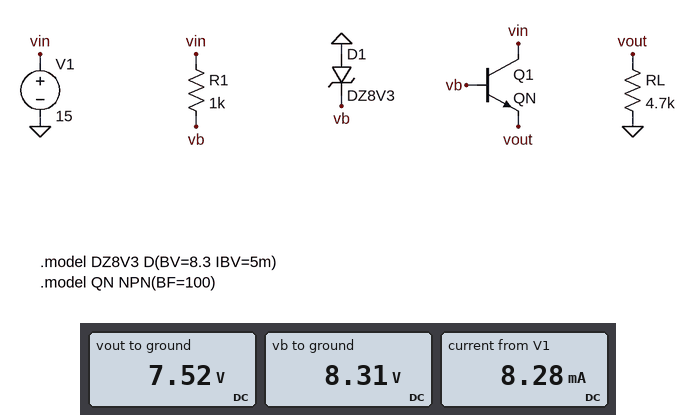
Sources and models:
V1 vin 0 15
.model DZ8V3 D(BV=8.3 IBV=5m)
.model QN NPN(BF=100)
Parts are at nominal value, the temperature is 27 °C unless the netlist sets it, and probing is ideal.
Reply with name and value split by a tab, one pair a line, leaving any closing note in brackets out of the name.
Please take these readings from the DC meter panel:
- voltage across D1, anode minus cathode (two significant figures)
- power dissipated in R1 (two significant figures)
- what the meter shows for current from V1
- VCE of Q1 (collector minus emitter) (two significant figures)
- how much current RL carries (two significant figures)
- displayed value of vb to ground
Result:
voltage across D1, anode minus cathode	-8.3 V
power dissipated in R1	45 mW
what the meter shows for current from V1	8.28 mA
VCE of Q1 (collector minus emitter)	7.5 V
how much current RL carries	1.6 mA
displayed value of vb to ground	8.31 V
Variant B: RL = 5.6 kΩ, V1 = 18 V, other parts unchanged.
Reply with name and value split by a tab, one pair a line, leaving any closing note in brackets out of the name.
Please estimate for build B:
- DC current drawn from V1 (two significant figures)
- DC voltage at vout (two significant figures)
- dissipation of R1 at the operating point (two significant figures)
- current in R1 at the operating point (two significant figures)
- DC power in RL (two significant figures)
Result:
DC current drawn from V1	11 mA
DC voltage at vout	7.5 V
dissipation of R1 at the operating point	94 mW
current in R1 at the operating point	9.7 mA
DC power in RL	10 mW
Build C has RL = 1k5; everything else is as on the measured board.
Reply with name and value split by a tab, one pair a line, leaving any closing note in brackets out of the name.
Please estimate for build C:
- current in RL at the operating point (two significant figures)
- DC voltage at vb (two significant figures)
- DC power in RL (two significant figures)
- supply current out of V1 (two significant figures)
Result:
current in RL at the operating point	5.0 mA
DC voltage at vb	8.3 V
DC power in RL	37 mW
supply current out of V1	12 mA
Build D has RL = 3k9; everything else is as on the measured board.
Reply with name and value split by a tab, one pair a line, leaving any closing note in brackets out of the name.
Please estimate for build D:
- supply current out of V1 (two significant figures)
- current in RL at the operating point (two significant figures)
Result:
supply current out of V1	8.6 mA
current in RL at the operating point	1.9 mA
